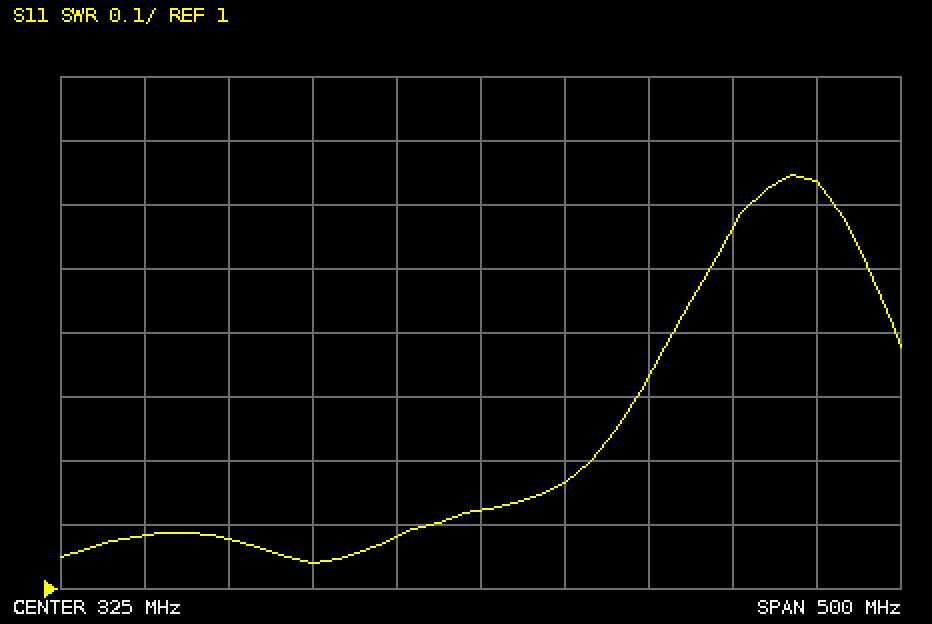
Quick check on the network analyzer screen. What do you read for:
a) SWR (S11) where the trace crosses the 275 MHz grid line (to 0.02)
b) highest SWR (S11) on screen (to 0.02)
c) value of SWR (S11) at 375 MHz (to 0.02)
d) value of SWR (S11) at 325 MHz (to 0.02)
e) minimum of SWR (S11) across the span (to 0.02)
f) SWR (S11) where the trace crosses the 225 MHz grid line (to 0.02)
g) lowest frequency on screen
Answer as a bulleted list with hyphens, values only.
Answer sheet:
- 1.08
- 1.64
- 1.16
- 1.12
- 1.04
- 1.04
- 75 MHz
